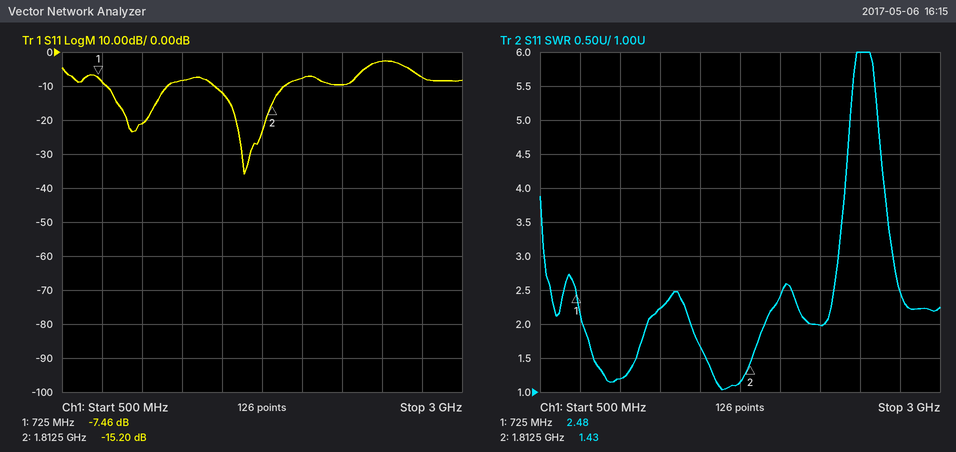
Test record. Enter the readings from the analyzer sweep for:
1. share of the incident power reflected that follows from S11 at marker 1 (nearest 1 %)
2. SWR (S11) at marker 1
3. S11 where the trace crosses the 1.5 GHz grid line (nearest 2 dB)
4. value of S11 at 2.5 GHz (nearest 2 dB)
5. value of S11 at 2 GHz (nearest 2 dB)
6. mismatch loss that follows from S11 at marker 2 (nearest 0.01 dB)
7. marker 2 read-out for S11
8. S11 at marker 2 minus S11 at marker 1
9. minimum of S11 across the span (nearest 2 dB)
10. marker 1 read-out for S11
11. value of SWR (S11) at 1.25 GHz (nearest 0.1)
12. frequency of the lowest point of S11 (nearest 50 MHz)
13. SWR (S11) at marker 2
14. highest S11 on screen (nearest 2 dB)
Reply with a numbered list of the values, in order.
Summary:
1. 18 %
2. 2.48
3. -12 dB
4. -2 dB
5. -8 dB
6. 0.13 dB
7. -15.20 dB
8. -7.74 dB
9. -36 dB
10. -7.46 dB
11. 2.2
12. 1.65 GHz
13. 1.43
14. -2 dB
